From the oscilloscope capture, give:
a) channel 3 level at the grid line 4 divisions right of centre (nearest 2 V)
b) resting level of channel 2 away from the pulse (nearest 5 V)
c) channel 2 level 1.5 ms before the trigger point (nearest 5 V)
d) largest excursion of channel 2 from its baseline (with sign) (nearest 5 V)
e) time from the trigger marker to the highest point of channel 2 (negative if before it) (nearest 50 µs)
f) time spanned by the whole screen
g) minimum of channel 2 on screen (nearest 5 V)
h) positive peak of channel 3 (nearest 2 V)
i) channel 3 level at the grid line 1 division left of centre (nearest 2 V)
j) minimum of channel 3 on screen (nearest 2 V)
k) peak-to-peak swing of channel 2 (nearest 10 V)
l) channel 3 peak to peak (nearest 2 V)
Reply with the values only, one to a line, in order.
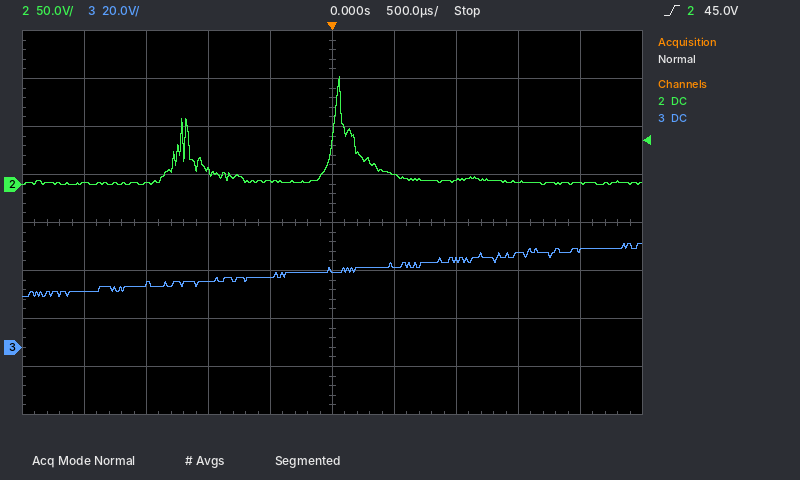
40 V
0 V
0 V
+110 V
+50 µs
5 ms
0 V
44 V
30 V
22 V
110 V
22 V
